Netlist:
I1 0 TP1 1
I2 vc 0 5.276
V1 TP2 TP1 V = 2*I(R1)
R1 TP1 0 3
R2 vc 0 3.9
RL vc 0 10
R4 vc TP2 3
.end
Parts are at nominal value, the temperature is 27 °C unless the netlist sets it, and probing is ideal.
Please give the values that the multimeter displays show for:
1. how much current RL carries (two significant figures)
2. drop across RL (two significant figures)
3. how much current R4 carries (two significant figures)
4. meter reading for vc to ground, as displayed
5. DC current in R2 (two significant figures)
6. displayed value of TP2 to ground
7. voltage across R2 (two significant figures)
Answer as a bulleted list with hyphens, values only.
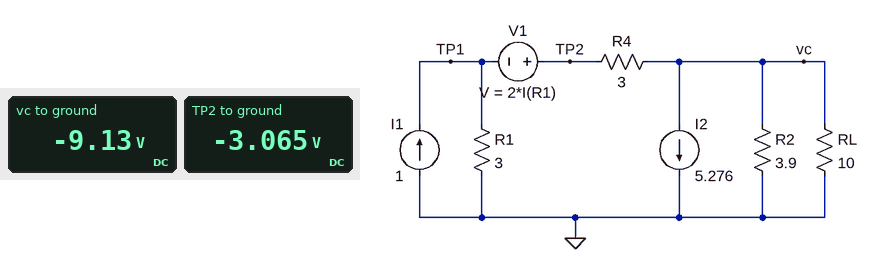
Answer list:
- 910 mA
- 9.1 V
- 2.0 A
- -9.13 V
- 2.3 A
- -3.065 V
- 9.1 V
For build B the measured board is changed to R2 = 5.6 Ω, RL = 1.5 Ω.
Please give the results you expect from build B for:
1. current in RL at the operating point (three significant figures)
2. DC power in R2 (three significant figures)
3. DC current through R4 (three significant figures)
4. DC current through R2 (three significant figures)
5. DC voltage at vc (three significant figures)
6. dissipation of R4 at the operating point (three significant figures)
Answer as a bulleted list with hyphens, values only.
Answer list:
- 3.15 A
- 3.98 W
- 1.29 A
- 843 mA
- -4.72 V
- 4.97 W
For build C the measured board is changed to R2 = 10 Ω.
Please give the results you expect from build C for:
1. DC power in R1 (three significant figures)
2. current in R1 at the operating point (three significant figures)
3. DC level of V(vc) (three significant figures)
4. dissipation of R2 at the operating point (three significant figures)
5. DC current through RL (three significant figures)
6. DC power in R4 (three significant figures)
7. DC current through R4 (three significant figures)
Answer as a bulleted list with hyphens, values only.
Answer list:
- 8.38 W
- 1.67 A
- -13.0 V
- 17.0 W
- 1.30 A
- 21.4 W
- 2.67 A
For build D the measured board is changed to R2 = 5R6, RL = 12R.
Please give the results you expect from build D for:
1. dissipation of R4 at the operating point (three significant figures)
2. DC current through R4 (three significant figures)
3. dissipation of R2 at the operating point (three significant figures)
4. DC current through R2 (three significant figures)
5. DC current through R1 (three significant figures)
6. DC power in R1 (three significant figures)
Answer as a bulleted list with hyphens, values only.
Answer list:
- 16.7 W
- 2.36 A
- 22.2 W
- 1.99 A
- 1.36 A
- 5.53 W
